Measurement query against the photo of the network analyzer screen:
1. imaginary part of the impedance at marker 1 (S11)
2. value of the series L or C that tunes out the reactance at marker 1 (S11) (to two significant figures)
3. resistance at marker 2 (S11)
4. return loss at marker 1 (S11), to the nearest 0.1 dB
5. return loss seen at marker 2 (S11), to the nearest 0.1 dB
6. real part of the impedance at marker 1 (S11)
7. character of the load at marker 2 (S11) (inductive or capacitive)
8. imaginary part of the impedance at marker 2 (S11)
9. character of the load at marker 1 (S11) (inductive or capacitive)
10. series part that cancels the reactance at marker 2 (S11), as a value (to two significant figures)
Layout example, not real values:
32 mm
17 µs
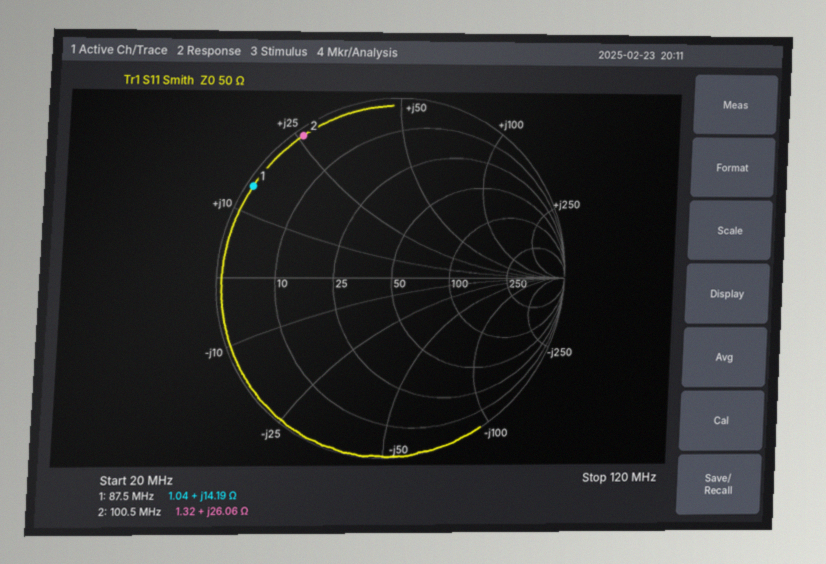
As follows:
+14.19 Ω
130 pF
1.32 Ω
0.3 dB
0.4 dB
1.04 Ω
inductive
+26.06 Ω
inductive
61 pF
